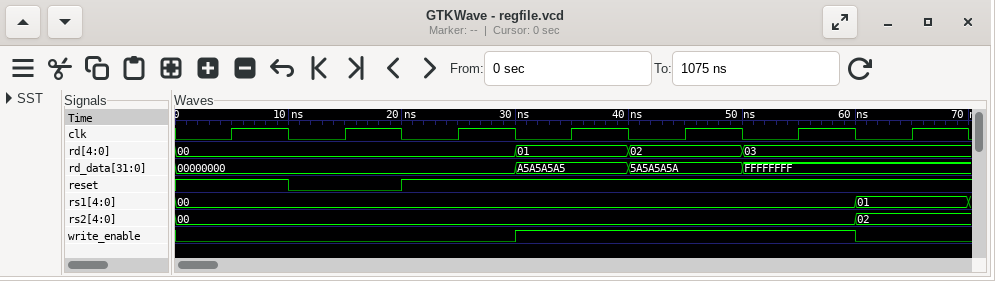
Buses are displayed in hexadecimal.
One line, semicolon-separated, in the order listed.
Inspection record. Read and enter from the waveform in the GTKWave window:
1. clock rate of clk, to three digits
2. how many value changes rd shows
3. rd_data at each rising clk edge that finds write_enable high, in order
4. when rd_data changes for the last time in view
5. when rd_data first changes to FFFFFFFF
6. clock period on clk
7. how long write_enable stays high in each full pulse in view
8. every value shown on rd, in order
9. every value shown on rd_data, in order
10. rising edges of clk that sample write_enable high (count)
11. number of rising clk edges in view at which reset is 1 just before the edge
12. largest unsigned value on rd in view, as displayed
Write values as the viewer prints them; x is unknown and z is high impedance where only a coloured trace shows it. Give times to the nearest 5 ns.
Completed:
100 MHz; 3; A5A5A5A5, 5A5A5A5A, FFFFFFFF; 50 ns; 50 ns; 10 ns; 30 ns; 00, 01, 02, 03; 00000000, A5A5A5A5, 5A5A5A5A, FFFFFFFF; 3; 6; 03
